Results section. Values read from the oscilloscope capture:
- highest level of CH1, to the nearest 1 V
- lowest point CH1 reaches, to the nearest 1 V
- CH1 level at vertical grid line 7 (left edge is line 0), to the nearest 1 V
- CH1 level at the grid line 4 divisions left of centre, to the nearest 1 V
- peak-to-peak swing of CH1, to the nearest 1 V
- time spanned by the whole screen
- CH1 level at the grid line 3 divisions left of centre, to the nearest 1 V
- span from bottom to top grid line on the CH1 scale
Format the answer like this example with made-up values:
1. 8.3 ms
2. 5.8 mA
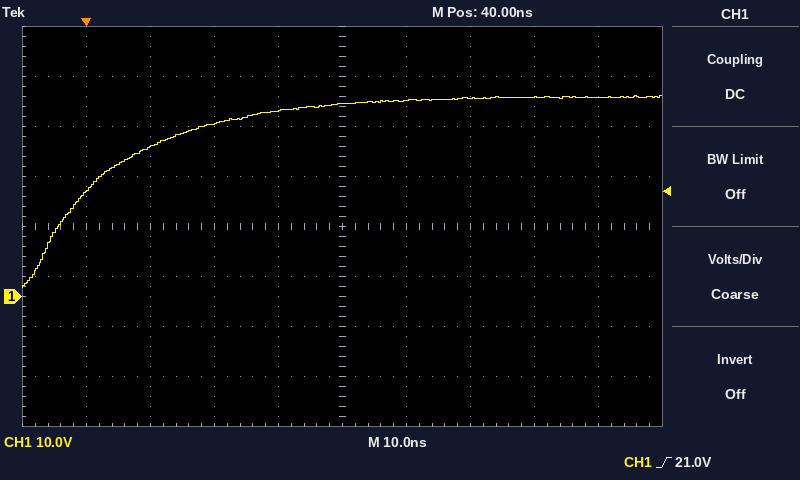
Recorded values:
1. 40 V
2. 2 V
3. 40 V
4. 21 V
5. 38 V
6. 100 ns
7. 30 V
8. 80 V
